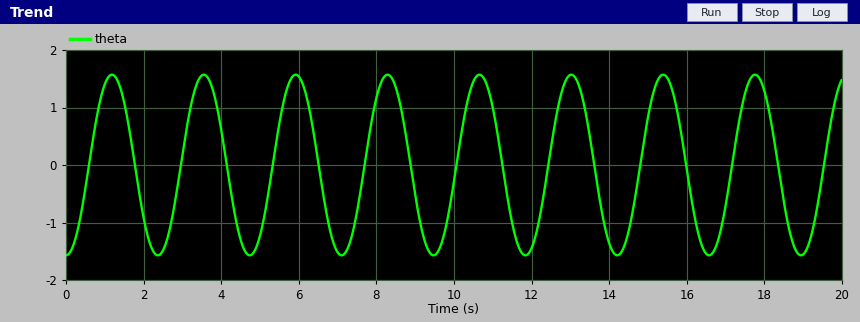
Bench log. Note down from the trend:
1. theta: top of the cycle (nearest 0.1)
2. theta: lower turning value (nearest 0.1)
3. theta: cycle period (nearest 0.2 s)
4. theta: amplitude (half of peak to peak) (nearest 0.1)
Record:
1.6
-1.6
2.4 s
1.6
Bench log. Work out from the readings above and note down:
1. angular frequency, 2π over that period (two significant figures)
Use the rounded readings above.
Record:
2.6 rad/s
